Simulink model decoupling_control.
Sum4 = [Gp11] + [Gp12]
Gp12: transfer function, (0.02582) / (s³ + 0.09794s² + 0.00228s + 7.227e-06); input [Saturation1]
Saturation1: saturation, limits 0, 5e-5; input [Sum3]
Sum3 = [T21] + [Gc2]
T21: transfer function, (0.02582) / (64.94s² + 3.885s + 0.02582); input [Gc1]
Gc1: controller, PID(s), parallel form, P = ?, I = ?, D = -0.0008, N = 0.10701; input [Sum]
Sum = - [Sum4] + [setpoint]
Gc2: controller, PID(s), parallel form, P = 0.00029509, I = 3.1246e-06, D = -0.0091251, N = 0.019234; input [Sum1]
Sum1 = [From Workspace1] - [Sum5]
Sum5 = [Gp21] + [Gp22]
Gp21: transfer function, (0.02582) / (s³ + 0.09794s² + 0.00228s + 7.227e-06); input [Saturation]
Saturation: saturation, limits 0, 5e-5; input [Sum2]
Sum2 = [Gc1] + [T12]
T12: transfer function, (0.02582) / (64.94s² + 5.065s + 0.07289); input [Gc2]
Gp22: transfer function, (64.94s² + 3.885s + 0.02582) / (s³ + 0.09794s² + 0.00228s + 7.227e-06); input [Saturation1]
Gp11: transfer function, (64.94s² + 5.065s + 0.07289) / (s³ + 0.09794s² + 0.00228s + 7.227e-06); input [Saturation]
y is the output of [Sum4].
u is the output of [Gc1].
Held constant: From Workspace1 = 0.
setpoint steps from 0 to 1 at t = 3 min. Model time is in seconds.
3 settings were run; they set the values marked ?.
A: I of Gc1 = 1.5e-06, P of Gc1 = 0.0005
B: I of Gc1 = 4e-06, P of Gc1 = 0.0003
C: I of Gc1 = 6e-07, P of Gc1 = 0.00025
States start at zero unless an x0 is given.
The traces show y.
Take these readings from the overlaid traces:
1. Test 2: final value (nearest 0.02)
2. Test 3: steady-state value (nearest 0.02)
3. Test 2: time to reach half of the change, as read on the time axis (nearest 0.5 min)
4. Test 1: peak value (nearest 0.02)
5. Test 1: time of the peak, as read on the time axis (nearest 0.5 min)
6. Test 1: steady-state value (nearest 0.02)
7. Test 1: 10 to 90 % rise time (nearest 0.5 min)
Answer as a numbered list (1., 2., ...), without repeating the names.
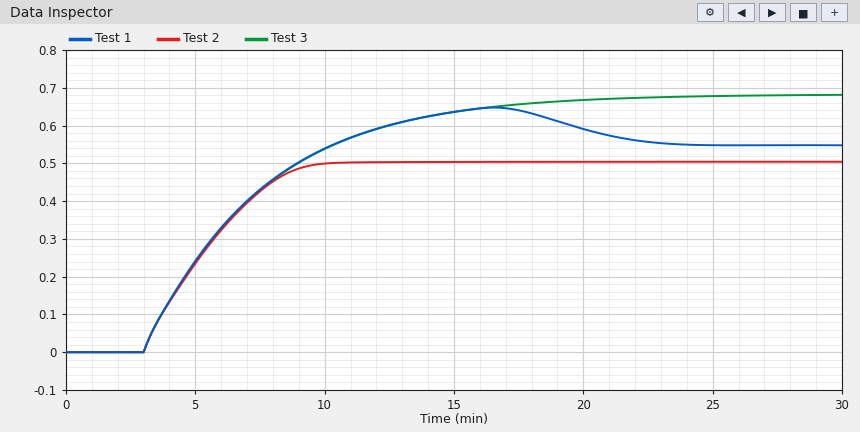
1. 0.50
2. 0.68
3. 5.0 min
4. 0.64
5. 16.5 min
6. 0.54
7. 5.5 min
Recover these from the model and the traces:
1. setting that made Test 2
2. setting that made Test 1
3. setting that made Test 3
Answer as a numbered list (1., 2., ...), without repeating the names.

1. C
2. A
3. B
